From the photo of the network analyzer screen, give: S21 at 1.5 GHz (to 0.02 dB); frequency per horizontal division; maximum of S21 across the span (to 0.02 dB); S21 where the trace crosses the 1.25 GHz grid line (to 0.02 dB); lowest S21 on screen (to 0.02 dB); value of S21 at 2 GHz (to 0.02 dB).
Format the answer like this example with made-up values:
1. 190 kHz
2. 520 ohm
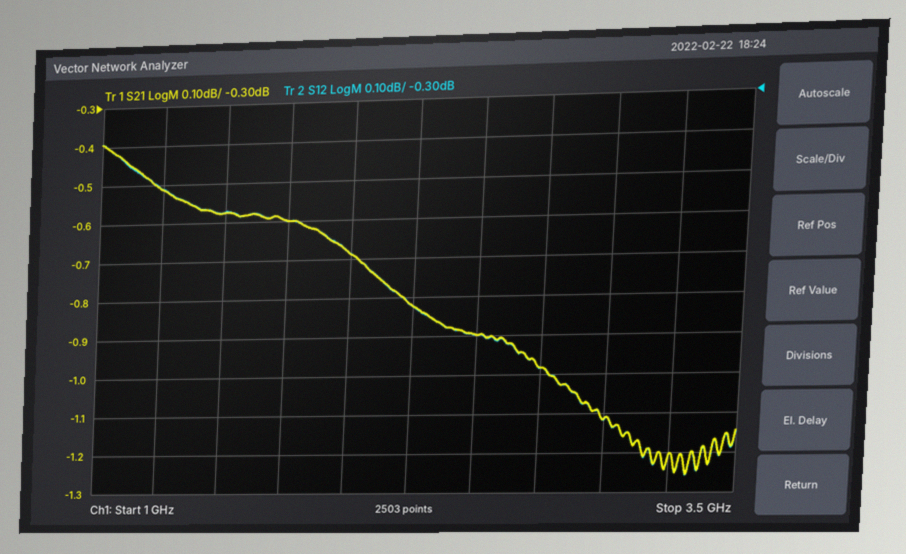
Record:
1. -0.58 dB
2. 250 MHz
3. -0.40 dB
4. -0.52 dB
5. -1.26 dB
6. -0.68 dB
